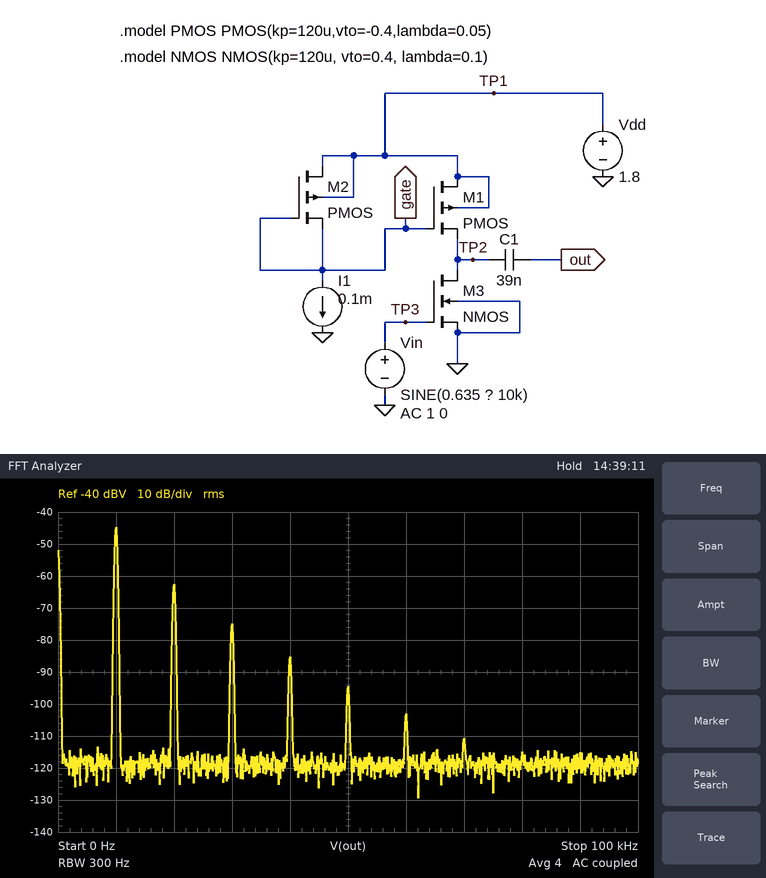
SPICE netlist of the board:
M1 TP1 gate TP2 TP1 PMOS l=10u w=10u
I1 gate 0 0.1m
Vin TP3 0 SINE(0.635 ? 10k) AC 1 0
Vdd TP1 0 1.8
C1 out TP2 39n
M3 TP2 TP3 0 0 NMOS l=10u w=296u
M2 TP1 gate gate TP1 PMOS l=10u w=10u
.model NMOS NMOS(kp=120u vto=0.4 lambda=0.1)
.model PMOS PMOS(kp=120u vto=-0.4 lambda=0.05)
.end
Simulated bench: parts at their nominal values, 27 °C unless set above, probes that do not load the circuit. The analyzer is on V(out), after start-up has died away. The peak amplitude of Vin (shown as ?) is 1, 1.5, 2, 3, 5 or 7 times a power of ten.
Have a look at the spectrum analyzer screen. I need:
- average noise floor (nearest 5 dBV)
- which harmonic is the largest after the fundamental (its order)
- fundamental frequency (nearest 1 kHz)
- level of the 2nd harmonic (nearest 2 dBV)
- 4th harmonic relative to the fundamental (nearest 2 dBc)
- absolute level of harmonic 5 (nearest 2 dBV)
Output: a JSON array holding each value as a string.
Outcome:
["-120 dBV", "2", "10 kHz", "-62 dBV", "-40 dBc", "-94 dBV"]
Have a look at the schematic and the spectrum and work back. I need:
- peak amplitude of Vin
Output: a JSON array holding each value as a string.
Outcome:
["700 µV"]
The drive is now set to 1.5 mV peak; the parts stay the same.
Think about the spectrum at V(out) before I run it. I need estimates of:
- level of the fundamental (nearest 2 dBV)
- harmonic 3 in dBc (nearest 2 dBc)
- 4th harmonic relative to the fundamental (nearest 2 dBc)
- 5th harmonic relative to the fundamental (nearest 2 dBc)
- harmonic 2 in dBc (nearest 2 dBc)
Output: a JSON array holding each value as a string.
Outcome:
["-34 dBV", "-16 dBc", "-34 dBc", "-30 dBc", "-8 dBc"]
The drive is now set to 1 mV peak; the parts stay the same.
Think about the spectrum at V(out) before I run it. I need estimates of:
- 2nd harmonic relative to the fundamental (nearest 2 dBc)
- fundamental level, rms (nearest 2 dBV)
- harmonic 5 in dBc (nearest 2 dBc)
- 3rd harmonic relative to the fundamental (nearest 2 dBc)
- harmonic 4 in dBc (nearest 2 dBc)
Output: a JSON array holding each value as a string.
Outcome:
["-12 dBc", "-40 dBV", "-30 dBc", "-18 dBc", "-24 dBc"]
